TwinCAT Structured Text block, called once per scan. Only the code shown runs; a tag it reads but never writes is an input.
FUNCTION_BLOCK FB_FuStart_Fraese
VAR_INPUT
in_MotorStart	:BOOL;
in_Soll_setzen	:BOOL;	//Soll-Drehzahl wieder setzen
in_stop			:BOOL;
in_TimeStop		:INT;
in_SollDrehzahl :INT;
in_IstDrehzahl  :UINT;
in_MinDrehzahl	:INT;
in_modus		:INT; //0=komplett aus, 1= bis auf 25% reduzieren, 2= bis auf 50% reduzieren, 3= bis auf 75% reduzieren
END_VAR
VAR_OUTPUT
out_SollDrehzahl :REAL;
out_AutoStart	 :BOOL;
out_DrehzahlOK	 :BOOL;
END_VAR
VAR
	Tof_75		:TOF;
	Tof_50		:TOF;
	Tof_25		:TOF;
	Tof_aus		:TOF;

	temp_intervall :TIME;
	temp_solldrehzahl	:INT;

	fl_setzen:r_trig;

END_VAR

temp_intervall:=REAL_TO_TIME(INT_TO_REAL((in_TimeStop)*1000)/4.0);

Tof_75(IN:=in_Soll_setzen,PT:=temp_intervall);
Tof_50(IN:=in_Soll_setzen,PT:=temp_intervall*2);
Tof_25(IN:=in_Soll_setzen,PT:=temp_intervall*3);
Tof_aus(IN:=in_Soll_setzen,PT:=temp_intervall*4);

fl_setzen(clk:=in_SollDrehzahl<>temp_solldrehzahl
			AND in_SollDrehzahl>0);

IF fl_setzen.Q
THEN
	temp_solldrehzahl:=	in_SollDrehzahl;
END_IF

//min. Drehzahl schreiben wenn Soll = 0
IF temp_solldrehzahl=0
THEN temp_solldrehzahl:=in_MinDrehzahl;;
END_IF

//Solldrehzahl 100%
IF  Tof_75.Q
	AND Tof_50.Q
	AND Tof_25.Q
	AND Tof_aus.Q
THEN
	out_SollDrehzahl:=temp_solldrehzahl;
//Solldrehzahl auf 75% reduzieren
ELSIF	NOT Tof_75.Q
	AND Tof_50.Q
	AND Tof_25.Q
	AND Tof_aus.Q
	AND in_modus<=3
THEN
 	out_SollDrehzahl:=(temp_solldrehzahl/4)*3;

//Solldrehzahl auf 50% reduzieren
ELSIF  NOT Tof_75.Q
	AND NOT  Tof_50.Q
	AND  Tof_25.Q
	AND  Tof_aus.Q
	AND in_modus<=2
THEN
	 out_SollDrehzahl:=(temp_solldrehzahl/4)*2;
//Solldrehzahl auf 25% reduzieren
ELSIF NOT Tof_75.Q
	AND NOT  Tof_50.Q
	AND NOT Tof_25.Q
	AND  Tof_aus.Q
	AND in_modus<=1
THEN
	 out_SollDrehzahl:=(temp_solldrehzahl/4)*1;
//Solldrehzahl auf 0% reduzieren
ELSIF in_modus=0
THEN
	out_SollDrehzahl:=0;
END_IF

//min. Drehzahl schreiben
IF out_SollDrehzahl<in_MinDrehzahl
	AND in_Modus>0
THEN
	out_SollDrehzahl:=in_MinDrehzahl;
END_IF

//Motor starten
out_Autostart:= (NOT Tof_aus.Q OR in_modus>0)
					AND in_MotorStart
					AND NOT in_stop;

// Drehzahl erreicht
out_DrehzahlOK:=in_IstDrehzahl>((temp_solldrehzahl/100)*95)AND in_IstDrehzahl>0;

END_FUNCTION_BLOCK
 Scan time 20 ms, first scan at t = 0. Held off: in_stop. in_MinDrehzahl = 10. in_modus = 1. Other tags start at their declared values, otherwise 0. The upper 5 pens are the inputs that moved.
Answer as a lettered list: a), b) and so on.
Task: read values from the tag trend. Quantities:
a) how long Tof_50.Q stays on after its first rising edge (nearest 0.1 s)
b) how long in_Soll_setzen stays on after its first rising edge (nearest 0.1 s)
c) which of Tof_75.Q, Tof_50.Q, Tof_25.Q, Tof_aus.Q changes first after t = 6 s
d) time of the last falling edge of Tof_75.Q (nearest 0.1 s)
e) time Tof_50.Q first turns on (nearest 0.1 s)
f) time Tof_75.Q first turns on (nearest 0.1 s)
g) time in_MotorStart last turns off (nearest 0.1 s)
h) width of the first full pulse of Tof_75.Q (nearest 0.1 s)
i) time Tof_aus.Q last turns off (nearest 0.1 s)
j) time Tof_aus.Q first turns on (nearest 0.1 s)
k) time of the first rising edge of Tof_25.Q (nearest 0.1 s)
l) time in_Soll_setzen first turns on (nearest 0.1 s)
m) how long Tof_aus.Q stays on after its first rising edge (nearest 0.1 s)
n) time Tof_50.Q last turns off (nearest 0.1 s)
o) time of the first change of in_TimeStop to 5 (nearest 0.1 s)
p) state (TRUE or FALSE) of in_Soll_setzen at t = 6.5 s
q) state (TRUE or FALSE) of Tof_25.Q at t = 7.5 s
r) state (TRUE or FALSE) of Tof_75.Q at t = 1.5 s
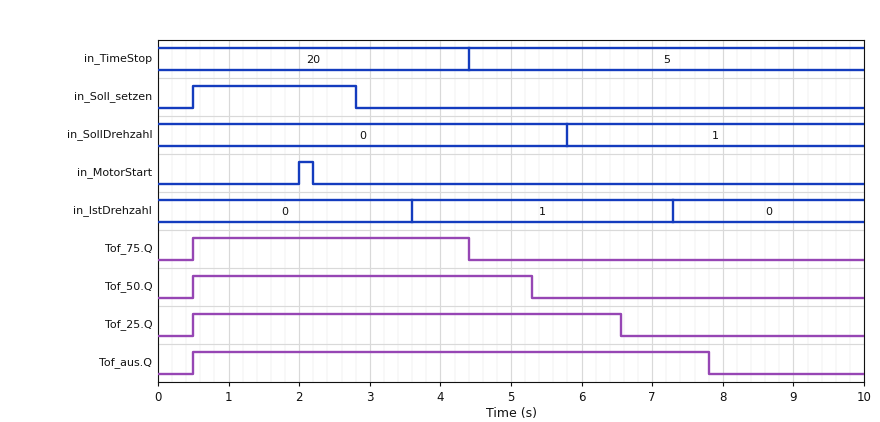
a) 4.8 s
b) 2.3 s
c) Tof_25.Q
d) 4.4 s
e) 0.5 s
f) 0.5 s
g) 2.2 s
h) 3.9 s
i) 7.8 s
j) 0.5 s
k) 0.5 s
l) 0.5 s
m) 7.3 s
n) 5.3 s
o) 4.4 s
p) FALSE
q) FALSE
r) TRUE
